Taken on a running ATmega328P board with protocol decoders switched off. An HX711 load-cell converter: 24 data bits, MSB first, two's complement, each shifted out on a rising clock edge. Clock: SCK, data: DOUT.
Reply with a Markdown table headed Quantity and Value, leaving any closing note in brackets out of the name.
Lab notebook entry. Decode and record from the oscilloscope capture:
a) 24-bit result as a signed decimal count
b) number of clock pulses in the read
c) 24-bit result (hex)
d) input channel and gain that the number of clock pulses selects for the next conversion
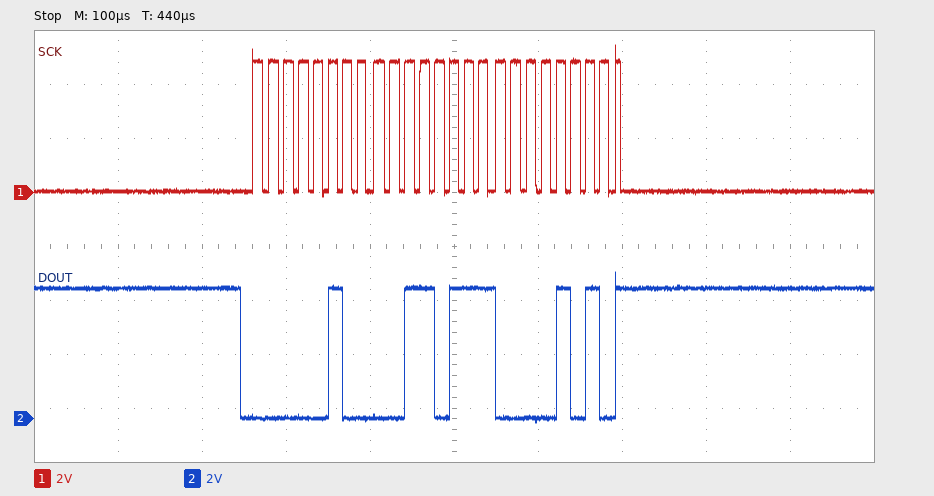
| Quantity | Value |
|---|---|
| 24-bit result as a signed decimal count | 276234 |
| number of clock pulses in the read | 25 |
| 24-bit result | 0x04370A |
| input channel and gain that the number of clock pulses selects for the next conversion | channel A, gain 128 |
